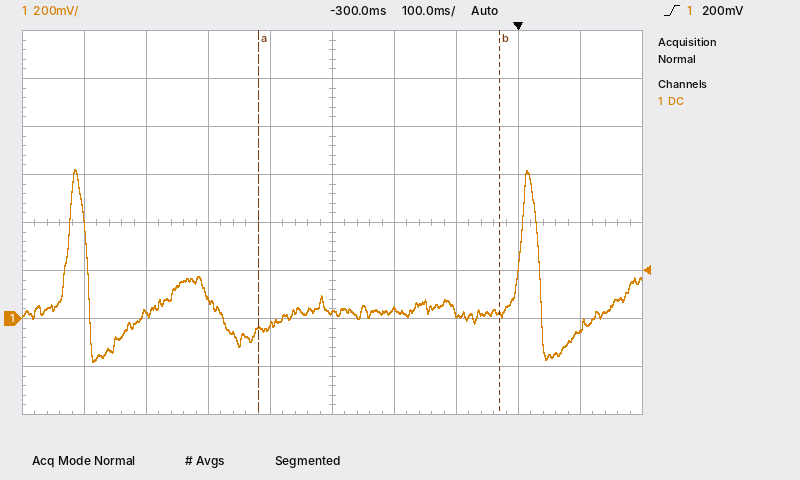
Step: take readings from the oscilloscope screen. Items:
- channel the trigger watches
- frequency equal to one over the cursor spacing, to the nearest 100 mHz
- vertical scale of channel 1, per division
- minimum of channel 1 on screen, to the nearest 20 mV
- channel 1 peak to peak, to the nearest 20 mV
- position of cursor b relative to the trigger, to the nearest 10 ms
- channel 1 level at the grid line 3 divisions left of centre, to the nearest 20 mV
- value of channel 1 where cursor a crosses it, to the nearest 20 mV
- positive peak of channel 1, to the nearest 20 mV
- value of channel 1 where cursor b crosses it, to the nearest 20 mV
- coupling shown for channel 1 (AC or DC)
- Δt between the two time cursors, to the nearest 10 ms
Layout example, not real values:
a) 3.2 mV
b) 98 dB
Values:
a) channel 1
b) 2.6 Hz
c) 200 mV
d) -180 mV
e) 800 mV
f) -30 ms
g) 20 mV
h) -40 mV
i) 620 mV
j) 20 mV
k) DC
l) 390 ms
